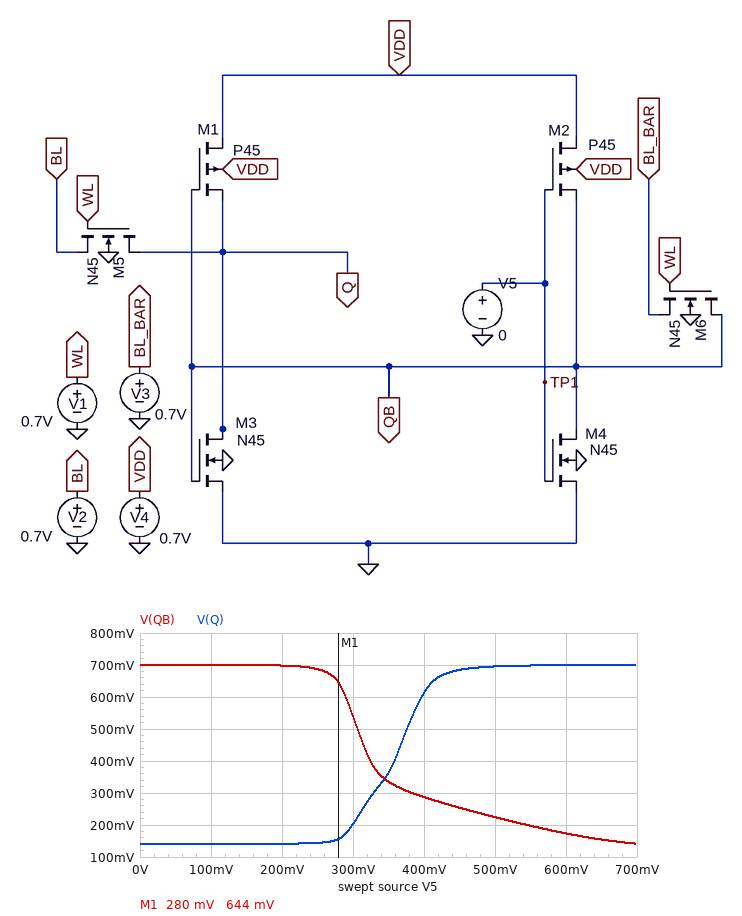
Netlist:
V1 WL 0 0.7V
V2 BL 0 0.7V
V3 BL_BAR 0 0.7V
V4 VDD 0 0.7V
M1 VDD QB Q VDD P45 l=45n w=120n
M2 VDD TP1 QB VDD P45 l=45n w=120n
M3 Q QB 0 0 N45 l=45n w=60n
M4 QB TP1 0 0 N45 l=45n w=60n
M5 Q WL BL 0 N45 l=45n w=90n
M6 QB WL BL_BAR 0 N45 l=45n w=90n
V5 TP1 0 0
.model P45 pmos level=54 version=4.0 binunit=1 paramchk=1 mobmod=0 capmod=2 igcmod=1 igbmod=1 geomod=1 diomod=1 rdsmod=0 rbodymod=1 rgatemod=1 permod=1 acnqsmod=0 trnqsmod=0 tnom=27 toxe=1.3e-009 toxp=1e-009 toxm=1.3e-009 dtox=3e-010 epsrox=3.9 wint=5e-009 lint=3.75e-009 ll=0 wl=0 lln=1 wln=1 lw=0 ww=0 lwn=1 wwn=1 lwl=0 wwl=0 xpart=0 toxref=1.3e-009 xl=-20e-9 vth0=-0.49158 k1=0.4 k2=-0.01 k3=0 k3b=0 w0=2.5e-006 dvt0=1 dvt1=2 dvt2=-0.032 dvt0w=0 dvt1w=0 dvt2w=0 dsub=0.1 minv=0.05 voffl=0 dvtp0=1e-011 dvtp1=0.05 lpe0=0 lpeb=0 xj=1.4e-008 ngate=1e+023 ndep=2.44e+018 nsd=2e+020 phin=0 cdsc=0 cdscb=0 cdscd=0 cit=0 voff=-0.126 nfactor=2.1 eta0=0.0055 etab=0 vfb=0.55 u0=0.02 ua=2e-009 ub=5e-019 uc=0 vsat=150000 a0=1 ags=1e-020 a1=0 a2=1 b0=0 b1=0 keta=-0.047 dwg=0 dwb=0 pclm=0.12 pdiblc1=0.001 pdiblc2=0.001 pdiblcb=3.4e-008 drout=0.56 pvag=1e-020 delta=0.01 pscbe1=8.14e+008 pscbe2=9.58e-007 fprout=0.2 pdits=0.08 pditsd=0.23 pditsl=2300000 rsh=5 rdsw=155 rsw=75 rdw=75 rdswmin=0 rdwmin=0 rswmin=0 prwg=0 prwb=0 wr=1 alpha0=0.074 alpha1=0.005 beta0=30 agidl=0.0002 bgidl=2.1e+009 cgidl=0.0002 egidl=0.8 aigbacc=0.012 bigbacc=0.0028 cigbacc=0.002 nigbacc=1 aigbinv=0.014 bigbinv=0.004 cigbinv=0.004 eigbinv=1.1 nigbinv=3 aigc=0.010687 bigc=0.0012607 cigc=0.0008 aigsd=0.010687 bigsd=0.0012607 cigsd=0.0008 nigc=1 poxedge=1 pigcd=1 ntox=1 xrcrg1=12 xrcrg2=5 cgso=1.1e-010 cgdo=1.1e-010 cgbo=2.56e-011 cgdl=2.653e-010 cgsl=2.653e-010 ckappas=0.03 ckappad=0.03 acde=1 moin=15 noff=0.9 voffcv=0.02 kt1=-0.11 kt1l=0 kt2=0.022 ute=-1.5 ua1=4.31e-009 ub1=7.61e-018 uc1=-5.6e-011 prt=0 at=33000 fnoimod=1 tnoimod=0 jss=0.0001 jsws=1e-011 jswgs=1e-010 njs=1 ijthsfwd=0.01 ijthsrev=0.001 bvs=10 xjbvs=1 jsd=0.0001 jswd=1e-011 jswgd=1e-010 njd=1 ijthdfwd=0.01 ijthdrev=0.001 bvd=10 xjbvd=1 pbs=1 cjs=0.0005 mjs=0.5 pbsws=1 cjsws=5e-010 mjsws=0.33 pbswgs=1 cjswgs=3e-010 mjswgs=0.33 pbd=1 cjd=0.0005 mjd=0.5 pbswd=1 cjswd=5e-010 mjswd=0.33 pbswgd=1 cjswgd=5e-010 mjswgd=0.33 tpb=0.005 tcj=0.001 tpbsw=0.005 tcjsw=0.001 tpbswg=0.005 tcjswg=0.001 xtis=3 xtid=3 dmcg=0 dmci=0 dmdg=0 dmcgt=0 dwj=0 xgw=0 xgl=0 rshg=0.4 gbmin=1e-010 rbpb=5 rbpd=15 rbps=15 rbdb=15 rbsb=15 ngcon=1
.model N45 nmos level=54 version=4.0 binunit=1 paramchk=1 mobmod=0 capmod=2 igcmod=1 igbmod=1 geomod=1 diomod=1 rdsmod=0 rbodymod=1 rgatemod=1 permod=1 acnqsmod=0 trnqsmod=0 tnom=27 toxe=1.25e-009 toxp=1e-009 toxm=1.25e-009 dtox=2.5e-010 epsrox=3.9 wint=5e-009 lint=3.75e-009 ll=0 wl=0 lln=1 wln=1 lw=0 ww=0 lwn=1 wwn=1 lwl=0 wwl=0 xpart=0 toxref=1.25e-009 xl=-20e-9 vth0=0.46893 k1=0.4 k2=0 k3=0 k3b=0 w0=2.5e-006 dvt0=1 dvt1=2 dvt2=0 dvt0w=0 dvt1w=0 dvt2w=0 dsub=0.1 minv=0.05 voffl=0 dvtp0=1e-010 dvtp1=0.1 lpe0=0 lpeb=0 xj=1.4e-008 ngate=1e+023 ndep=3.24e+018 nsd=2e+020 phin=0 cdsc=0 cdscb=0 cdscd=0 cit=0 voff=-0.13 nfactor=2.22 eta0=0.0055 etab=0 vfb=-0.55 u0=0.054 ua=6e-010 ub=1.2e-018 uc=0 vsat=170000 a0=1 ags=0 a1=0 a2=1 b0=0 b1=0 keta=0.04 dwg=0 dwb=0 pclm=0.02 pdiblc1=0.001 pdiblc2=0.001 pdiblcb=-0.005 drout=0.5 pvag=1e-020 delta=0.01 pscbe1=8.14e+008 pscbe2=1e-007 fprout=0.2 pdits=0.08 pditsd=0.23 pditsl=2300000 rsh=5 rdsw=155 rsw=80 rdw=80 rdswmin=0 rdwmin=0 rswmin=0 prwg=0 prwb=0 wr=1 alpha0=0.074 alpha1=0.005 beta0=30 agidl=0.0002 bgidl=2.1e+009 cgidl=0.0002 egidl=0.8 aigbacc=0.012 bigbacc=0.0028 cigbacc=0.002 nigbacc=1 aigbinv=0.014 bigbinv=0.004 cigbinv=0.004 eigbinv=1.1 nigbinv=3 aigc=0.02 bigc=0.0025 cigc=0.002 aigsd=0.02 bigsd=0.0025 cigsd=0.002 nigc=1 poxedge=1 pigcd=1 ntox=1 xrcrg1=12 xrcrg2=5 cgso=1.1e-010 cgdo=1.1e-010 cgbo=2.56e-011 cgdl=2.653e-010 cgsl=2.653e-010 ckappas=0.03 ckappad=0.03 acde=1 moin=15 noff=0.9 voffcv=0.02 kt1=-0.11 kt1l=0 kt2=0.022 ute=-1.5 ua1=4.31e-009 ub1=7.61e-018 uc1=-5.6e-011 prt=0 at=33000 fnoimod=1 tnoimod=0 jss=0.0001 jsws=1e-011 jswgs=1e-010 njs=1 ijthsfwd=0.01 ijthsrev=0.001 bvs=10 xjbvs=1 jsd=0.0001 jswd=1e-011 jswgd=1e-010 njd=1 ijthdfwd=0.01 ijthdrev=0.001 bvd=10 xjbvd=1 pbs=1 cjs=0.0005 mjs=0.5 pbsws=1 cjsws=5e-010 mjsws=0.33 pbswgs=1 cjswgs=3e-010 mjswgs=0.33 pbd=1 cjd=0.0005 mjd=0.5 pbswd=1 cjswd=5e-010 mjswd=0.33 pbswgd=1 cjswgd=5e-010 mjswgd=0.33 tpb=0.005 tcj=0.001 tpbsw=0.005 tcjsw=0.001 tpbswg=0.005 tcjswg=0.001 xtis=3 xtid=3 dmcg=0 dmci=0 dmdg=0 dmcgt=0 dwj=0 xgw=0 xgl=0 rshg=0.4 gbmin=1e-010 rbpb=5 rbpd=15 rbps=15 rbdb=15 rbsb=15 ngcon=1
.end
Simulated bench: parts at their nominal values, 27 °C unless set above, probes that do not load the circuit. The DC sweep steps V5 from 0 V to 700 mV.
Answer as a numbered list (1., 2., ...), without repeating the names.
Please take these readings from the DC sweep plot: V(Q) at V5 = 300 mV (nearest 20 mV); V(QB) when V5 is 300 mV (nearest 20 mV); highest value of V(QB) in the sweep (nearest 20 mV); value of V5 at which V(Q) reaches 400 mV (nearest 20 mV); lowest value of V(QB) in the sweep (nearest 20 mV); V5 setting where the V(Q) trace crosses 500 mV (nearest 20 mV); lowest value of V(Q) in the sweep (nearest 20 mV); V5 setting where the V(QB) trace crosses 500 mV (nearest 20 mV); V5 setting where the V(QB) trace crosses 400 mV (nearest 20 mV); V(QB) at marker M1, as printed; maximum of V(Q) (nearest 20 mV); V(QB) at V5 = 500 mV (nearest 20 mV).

1. 200 mV
2. 540 mV
3. 700 mV
4. 360 mV
5. 140 mV
6. 380 mV
7. 140 mV
8. 300 mV
9. 320 mV
10. 644 mV
11. 700 mV
12. 220 mV
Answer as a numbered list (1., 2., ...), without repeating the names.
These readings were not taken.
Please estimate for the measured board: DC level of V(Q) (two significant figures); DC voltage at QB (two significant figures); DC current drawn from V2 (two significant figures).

1. 140 mV
2. 700 mV
3. 18 µA
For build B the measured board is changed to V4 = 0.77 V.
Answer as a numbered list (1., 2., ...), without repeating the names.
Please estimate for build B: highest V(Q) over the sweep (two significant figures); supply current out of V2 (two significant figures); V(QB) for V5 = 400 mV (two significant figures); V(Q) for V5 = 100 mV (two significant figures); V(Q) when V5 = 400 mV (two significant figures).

1. 770 mV
2. 21 µA
3. 300 mV
4. 130 mV
5. 730 mV
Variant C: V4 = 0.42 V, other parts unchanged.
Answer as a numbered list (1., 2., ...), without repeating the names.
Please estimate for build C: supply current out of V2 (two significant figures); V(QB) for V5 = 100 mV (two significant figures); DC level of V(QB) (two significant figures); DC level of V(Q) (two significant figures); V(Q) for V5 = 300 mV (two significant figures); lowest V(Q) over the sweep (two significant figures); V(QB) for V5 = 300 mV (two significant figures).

1. 1.8 µA
2. 430 mV
3. 420 mV
4. 270 mV
5. 320 mV
6. 260 mV
7. 350 mV
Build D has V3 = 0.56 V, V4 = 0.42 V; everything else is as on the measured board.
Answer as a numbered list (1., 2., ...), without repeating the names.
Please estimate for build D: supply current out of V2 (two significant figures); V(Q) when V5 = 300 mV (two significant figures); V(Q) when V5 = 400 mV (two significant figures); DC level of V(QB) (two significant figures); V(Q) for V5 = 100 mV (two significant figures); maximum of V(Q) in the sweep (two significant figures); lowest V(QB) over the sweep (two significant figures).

1. 1.8 µA
2. 330 mV
3. 370 mV
4. 420 mV
5. 270 mV
6. 430 mV
7. 130 mV
